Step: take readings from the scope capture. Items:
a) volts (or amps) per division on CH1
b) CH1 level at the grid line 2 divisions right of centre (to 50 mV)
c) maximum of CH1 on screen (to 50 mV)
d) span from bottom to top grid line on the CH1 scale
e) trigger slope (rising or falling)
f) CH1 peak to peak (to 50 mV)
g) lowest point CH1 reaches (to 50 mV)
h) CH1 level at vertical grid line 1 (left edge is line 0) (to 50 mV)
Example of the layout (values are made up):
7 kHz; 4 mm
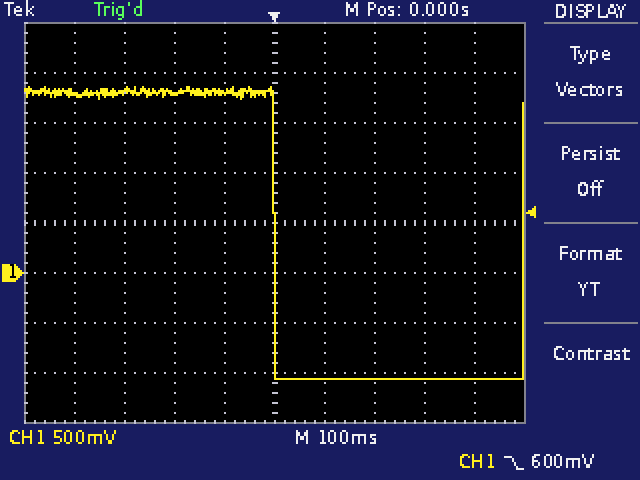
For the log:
500 mV; -1.05 V; 1.85 V; 4 V; falling; 2.90 V; -1.05 V; 1.80 V
